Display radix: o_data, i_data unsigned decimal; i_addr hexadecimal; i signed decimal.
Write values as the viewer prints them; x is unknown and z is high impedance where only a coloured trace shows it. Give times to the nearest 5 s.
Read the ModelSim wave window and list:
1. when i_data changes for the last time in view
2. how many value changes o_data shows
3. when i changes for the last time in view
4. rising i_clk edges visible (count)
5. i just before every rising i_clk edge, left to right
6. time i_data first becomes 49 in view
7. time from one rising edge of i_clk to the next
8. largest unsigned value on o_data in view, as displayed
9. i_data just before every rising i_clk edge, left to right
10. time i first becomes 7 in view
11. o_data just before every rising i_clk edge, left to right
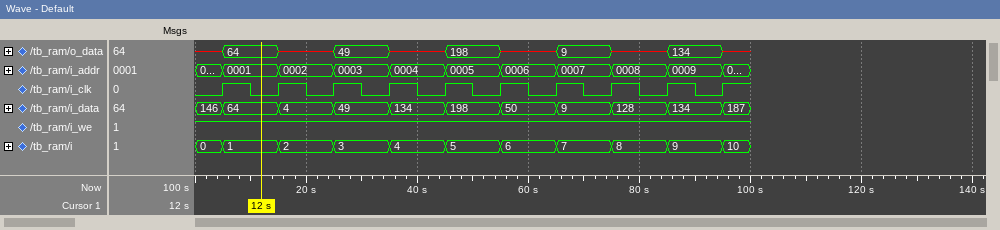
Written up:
95 s
10
95 s
10
0, 1, 2, 3, 4, 5, 6, 7, 8, 9
25 s
10 s
198
146, 64, 4, 49, 134, 198, 50, 9, 128, 134
65 s
x, 64, x, 49, x, 198, x, 9, x, 134
